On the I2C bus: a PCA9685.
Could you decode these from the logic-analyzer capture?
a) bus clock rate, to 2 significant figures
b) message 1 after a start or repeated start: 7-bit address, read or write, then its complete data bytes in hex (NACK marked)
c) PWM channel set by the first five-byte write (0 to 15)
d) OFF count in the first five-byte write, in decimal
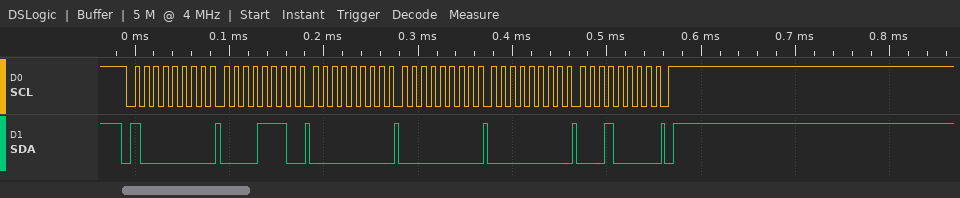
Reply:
100 kHz
0x40 write: 0E 00 00 00 10
2
4096
